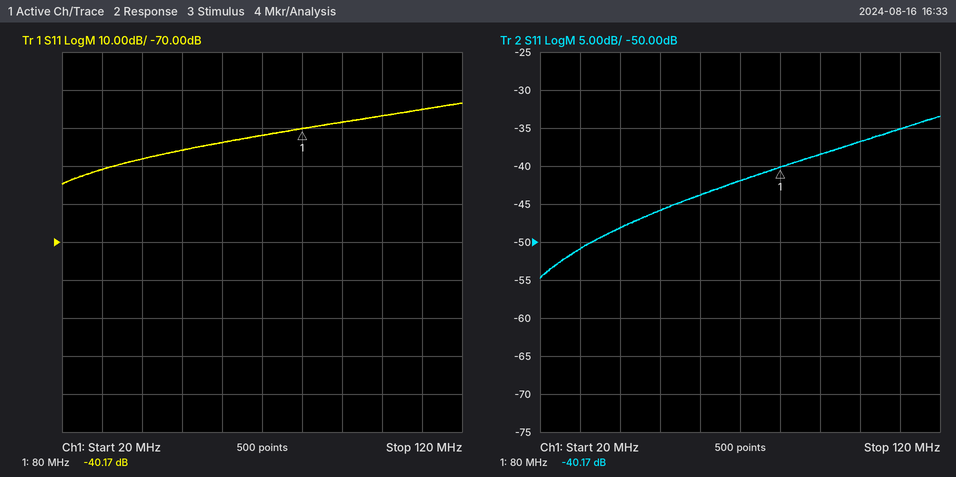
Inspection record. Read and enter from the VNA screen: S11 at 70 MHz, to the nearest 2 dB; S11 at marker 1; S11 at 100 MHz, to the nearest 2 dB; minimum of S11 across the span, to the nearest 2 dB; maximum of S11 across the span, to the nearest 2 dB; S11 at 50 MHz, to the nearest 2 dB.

-42 dB
-40.17 dB
-36 dB
-54 dB
-34 dB
-46 dB
